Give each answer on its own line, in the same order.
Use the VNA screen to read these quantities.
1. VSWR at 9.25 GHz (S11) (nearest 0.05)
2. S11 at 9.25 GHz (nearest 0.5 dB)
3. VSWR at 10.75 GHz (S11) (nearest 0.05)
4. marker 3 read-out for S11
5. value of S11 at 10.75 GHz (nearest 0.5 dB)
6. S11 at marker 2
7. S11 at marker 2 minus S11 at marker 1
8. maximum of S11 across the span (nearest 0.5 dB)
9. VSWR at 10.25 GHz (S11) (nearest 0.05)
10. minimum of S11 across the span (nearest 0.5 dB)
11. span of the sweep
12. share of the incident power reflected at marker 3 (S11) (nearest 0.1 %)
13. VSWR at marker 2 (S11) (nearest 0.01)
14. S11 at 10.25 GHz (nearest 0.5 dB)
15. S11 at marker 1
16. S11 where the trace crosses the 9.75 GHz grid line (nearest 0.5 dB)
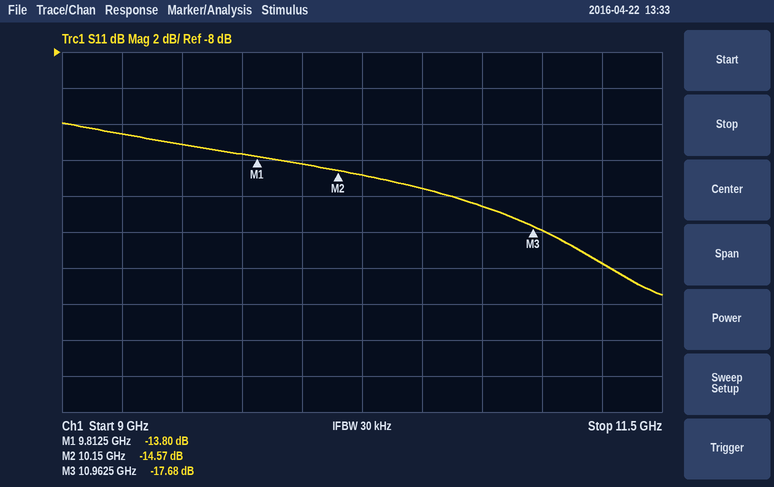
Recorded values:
1.60
-12.5 dB
1.35
-17.68 dB
-16.5 dB
-14.57 dB
-0.77 dB
-12.0 dB
1.45
-21.5 dB
2.5 GHz
1.7 %
1.46
-15.0 dB
-13.80 dB
-13.5 dB
